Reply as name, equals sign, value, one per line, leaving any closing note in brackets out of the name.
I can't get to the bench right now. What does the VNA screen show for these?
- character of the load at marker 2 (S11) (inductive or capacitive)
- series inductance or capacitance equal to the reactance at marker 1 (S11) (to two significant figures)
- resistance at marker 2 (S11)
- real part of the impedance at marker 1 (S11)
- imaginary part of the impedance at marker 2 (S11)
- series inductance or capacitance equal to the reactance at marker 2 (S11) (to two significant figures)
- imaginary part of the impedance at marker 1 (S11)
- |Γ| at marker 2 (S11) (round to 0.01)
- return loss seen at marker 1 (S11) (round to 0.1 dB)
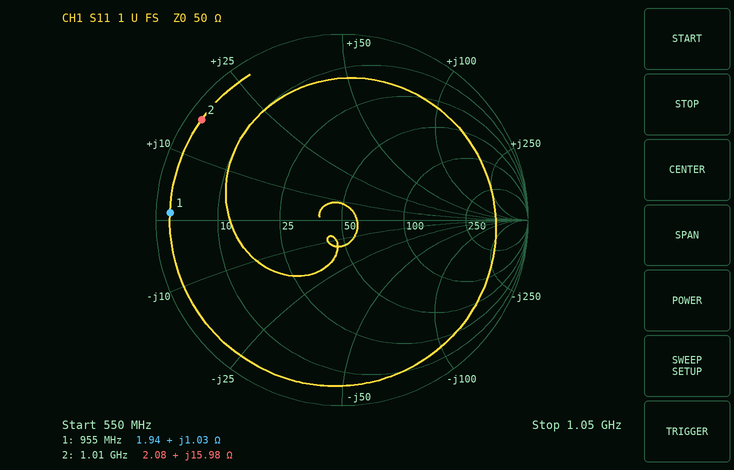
character of the load at marker 2 (S11) = inductive
series inductance or capacitance equal to the reactance at marker 1 (S11) = 170 pH
resistance at marker 2 = 2.08 Ω
real part of the impedance at marker 1 = 1.94 Ω
imaginary part of the impedance at marker 2 = +15.98 Ω
series inductance or capacitance equal to the reactance at marker 2 (S11) = 2.5 nH
imaginary part of the impedance at marker 1 = +1.03 Ω
|Γ| at marker 2 (S11) = 0.93
return loss seen at marker 1 (S11) = 0.7 dB
